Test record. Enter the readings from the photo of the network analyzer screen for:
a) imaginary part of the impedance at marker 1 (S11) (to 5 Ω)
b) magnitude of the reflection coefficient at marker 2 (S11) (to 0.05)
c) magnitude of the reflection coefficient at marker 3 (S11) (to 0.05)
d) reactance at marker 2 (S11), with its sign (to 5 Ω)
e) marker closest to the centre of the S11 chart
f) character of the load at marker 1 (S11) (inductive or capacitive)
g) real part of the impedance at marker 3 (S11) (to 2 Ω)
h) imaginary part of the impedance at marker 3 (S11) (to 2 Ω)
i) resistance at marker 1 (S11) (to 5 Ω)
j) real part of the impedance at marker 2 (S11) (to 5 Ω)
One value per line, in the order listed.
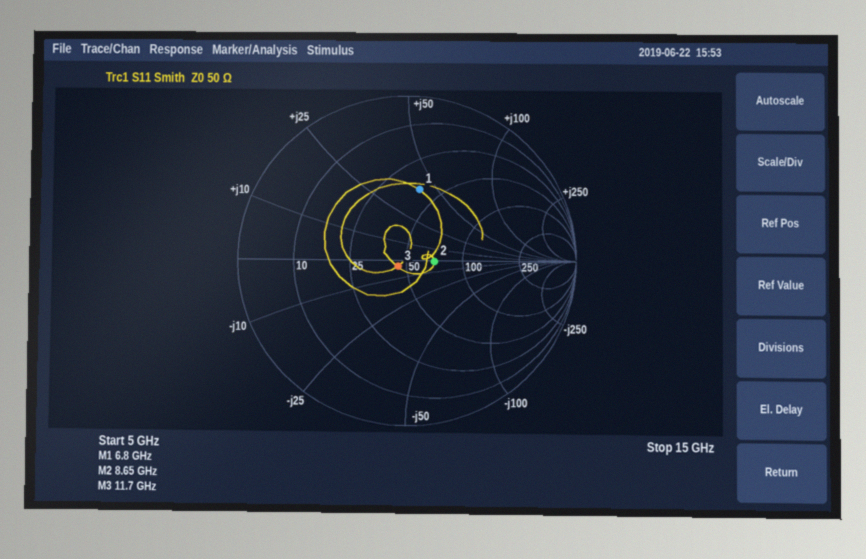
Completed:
+40 Ω
0.15
0.05
0 Ω
marker 3
inductive
46 Ω
-4 Ω
40 Ω
70 Ω
